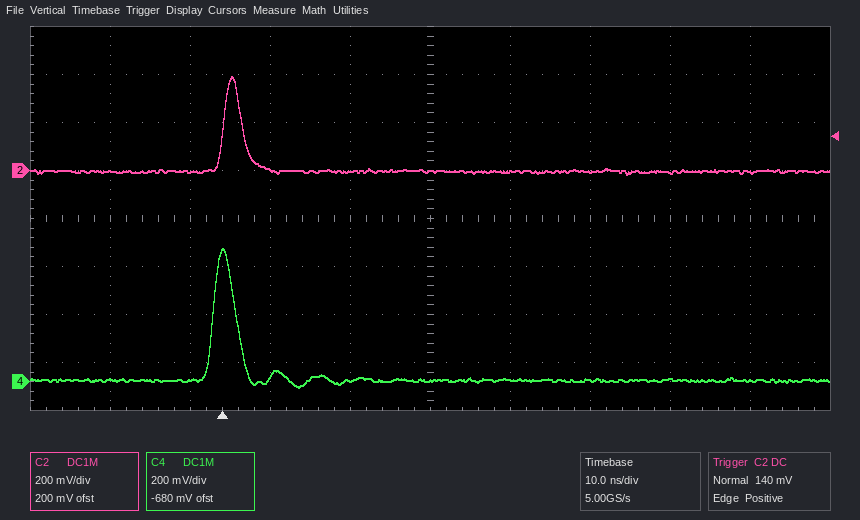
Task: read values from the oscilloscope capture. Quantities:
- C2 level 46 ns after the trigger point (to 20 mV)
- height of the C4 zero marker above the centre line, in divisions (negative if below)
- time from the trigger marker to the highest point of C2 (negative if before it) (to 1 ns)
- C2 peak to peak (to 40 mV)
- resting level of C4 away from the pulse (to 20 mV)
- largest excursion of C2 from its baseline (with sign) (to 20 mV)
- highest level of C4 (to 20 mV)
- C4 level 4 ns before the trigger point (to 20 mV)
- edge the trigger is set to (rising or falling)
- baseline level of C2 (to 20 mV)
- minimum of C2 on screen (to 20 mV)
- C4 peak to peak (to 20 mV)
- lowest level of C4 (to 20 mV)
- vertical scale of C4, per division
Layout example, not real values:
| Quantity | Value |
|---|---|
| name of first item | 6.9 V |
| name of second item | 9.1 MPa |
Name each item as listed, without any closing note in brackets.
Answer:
| Quantity | Value |
|---|---|
| C2 level 46 ns after the trigger point | 0 mV |
| height of the C4 zero marker above the centre line, in divisions | -3.4 div |
| time from the trigger marker to the highest point of C2 (negative if before it) | +1 ns |
| C2 peak to peak | 400 mV |
| resting level of C4 away from the pulse | 0 mV |
| largest excursion of C2 from its baseline (with sign) | +400 mV |
| highest level of C4 | 560 mV |
| C4 level 4 ns before the trigger point | 0 mV |
| edge the trigger is set to | rising |
| baseline level of C2 | 0 mV |
| minimum of C2 on screen | -20 mV |
| C4 peak to peak | 580 mV |
| lowest level of C4 | -20 mV |
| vertical scale of C4, per division | 200 mV |
